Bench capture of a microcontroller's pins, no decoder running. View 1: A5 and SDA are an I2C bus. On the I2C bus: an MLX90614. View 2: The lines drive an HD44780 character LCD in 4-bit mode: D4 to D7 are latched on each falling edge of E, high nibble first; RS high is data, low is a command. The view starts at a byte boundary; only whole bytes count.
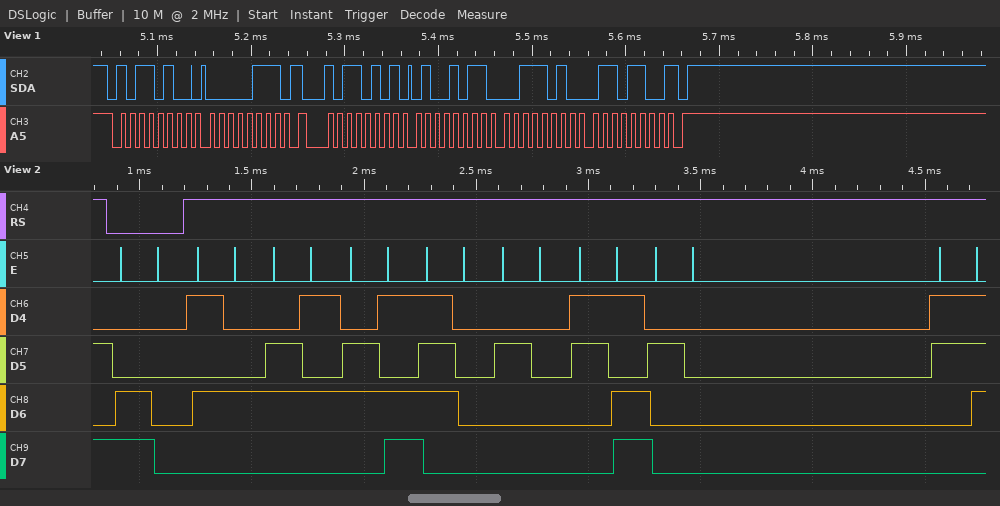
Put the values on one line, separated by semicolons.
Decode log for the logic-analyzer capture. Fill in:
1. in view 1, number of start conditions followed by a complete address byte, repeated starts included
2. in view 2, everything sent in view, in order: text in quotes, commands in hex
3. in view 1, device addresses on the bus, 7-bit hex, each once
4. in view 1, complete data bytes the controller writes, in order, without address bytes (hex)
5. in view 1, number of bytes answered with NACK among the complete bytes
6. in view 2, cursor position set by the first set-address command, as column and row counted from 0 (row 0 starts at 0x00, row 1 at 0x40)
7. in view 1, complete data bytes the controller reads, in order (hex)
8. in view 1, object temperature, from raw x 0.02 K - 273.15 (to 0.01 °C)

2; 0xC0 "Temp = 7"; 0x5A; 07; 1; column 0, row 1; 4B 3A 6C; 25.31 °C
